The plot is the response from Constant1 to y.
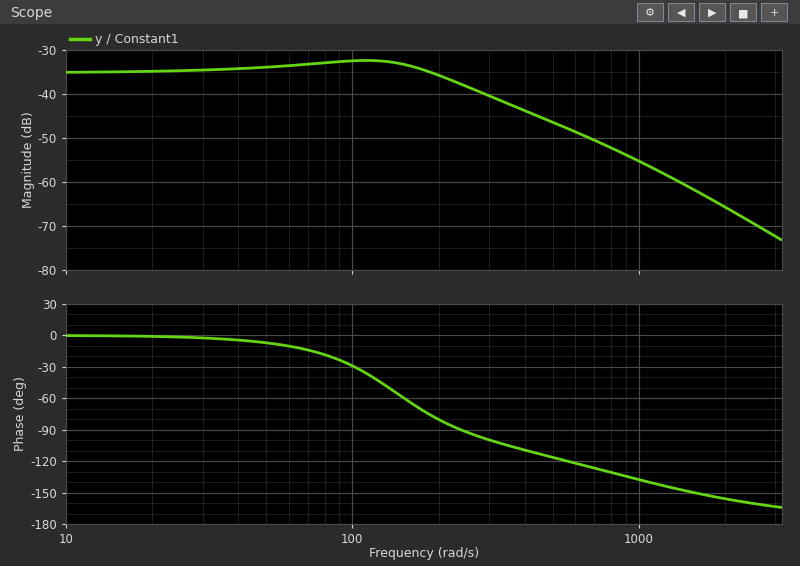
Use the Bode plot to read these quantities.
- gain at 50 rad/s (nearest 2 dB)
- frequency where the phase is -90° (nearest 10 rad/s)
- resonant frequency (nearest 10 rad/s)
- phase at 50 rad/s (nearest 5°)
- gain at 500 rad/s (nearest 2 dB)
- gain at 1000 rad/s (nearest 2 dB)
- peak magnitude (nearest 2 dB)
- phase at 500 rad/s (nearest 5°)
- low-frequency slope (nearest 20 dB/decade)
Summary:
-34 dB
240 rad/s
110 rad/s
-5°
-46 dB
-56 dB
-32 dB
-115°
0 dB/decade
